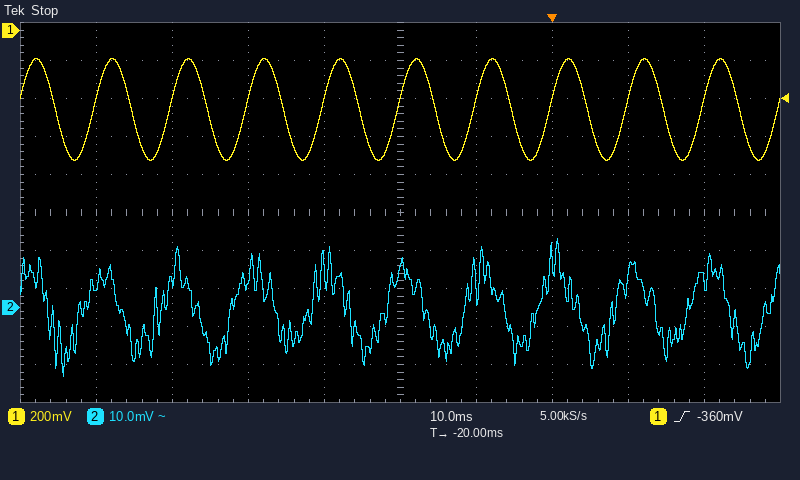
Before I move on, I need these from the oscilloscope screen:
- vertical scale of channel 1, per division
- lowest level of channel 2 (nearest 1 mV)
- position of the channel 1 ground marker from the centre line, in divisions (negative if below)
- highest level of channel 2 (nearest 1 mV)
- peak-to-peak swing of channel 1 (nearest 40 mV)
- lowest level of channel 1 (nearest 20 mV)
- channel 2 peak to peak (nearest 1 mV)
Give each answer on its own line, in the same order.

200 mV
-18 mV
+4.8 div
18 mV
520 mV
-680 mV
36 mV
